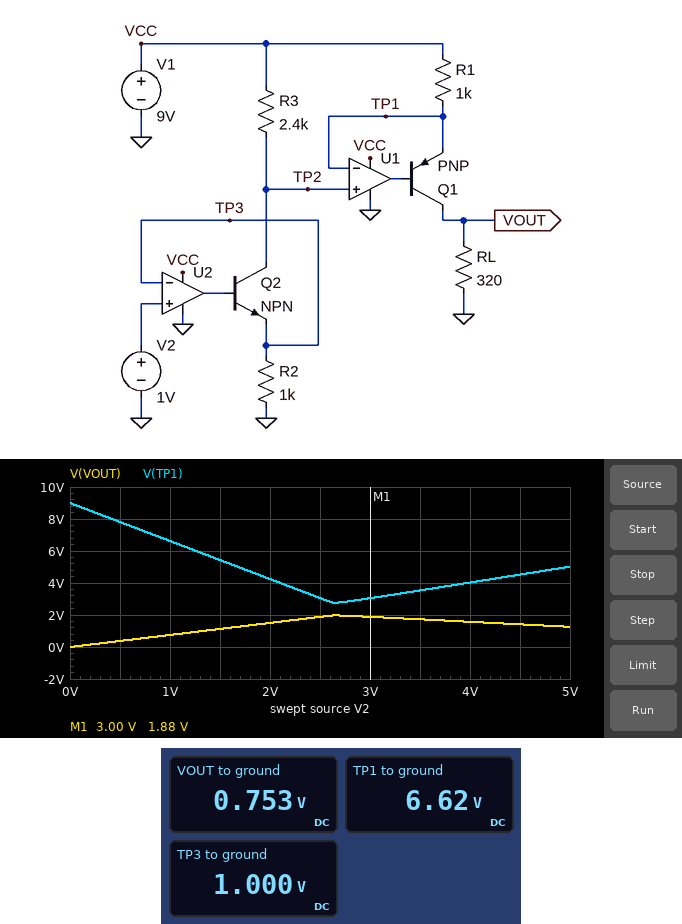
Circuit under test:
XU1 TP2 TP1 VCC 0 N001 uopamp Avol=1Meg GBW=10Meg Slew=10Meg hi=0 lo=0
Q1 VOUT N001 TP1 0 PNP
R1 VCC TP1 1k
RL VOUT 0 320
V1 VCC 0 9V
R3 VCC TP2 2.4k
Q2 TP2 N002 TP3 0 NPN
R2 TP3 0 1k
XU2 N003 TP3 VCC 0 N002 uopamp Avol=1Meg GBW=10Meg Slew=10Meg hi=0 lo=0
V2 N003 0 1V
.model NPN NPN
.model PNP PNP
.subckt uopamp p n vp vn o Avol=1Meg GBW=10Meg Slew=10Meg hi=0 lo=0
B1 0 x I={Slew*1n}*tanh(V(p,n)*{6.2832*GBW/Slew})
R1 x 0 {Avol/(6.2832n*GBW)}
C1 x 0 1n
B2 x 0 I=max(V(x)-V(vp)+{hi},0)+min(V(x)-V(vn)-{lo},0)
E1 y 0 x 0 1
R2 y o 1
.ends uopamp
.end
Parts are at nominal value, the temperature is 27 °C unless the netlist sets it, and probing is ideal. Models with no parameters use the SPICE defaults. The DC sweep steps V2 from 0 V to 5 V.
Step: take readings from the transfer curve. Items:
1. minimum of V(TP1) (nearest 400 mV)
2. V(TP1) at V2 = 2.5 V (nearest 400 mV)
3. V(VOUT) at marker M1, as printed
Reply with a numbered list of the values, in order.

1. 2.8 V
2. 3.2 V
3. 1.88 V
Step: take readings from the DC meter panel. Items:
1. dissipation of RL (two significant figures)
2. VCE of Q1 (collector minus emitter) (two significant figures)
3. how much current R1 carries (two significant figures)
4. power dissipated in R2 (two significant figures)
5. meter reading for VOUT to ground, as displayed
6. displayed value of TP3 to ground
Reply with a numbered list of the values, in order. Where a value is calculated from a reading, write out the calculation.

1. (753 mV)^2 / 320 Ω = 1.8 mW
2. 753 mV - 6.62 V = -5.9 V
3. (9 V - 6.62 V) / 1 kΩ = 2.4 mA
4. (1 V)^2 / 1 kΩ = 1.0 mW
5. 0.753 V
6. 1.000 V
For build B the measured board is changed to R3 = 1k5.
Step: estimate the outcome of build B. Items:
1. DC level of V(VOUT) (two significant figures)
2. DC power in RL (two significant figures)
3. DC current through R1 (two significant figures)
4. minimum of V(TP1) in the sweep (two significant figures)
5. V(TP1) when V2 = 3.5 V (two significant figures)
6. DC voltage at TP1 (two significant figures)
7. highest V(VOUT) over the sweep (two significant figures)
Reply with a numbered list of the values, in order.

1. 470 mV
2. 690 µW
3. 1.5 mA
4. 3.7 V
5. 3.8 V
6. 7.5 V
7. 1.7 V
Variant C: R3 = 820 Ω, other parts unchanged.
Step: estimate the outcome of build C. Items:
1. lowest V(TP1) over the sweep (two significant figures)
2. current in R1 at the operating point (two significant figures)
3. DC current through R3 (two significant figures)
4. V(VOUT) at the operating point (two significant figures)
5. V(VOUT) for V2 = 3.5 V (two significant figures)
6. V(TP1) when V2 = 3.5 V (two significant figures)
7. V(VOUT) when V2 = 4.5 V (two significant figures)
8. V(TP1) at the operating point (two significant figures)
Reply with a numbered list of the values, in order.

1. 5.0 V
2. 810 µA
3. 990 µA
4. 260 mV
5. 900 mV
6. 6.2 V
7. 1.2 V
8. 8.2 V
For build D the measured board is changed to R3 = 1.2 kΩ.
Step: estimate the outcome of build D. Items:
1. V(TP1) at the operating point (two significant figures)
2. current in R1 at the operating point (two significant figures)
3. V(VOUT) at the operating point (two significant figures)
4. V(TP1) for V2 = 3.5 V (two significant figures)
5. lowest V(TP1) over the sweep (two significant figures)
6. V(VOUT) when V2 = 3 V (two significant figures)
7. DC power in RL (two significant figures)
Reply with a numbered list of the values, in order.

1. 7.8 V
2. 1.2 mA
3. 380 mV
4. 4.8 V
5. 4.2 V
6. 1.1 V
7. 440 µW
